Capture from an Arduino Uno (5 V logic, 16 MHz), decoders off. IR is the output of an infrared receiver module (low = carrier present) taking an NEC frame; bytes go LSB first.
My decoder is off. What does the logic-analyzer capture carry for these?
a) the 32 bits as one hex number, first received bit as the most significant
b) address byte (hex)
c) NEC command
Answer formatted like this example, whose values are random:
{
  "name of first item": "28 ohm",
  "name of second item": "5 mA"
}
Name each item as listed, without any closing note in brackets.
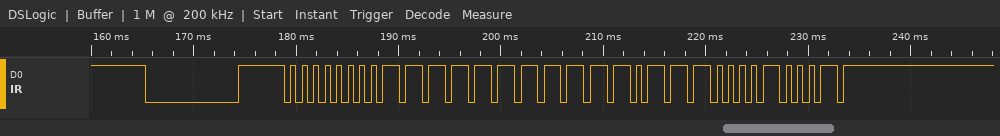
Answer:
{
  "the 32 bits as one hex number, first received bit as the most significant": "0x00FFEE11",
  "address byte": "0x00",
  "NEC command": "0x77"
}
